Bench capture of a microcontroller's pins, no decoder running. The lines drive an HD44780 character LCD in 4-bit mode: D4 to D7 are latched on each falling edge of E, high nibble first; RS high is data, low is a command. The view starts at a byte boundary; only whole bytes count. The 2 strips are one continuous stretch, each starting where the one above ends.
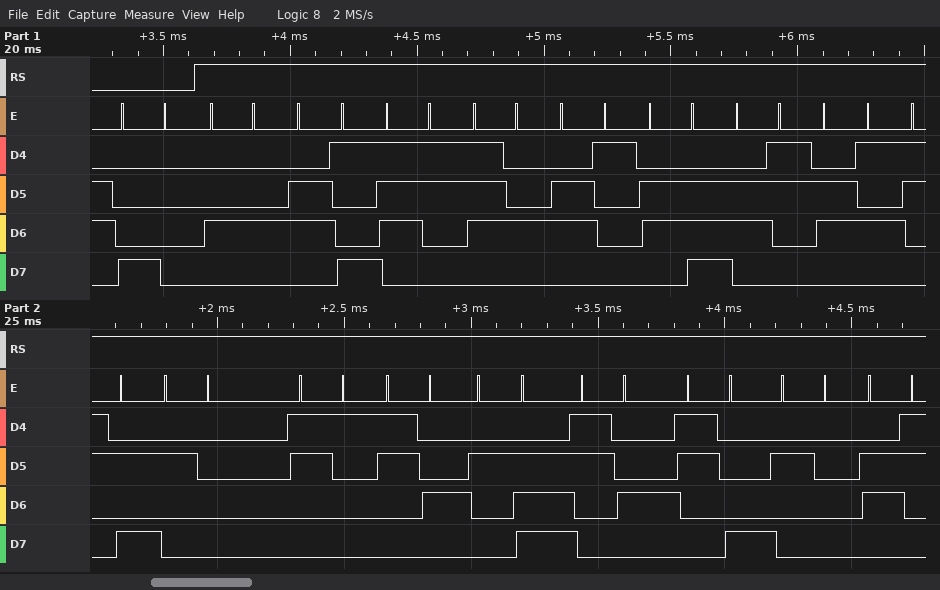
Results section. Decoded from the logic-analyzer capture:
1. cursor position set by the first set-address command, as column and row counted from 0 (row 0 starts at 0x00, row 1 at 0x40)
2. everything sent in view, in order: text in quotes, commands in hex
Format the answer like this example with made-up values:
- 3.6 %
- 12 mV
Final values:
- column 0, row 0
- 0x80 "Distance: 14.48 c"
